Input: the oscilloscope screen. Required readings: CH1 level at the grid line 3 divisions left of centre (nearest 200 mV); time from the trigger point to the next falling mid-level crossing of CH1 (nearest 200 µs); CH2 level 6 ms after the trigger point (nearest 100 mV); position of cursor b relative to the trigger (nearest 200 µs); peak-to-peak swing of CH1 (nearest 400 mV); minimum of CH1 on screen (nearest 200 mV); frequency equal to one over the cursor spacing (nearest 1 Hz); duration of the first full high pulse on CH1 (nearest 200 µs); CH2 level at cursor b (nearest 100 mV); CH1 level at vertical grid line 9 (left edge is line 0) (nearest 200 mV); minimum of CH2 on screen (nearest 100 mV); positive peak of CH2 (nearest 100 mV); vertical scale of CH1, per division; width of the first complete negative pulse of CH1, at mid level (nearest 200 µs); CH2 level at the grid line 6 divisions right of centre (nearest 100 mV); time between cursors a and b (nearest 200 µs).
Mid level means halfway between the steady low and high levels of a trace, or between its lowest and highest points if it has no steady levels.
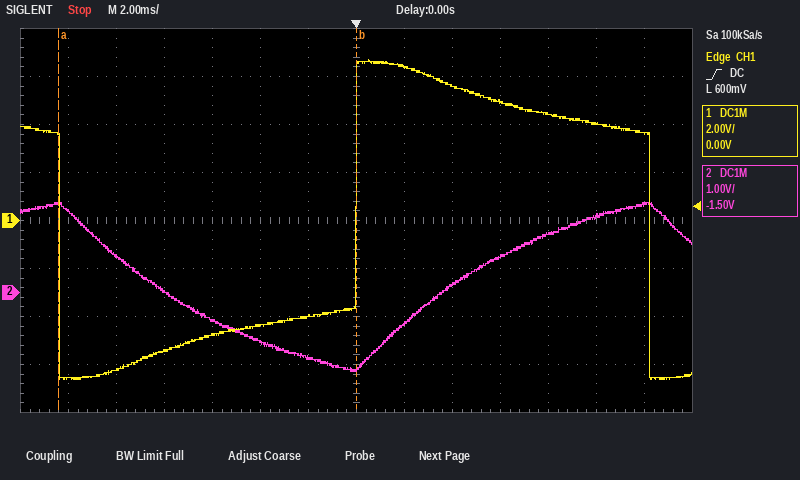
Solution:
-4.8 V
12.2 ms
700 mV
0.0 ms
13.2 V
-6.6 V
81 Hz
12.2 ms
-1.6 V
5.6 V
-1.6 V
1.9 V
2 V
12.4 ms
1.8 V
12.4 ms
